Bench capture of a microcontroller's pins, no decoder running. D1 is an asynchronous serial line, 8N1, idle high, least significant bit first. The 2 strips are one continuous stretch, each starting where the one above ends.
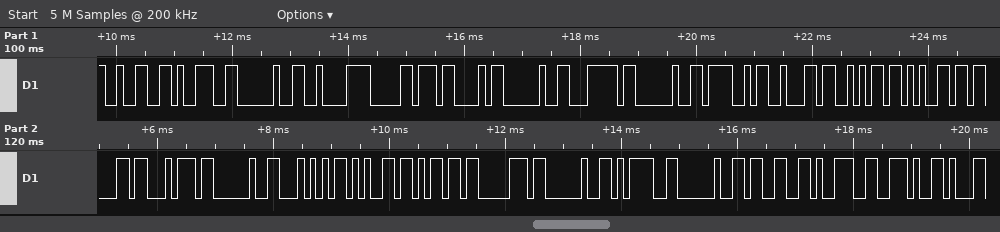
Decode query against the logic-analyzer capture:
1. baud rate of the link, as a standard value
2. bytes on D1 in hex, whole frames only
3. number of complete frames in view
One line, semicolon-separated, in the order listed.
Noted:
9600 baud; 0x32 0x39 0x20 0xC2 0xB0 0x43 0x20 0x7C 0x20 0x4F 0x62 0x6A 0x65 0x63 0x74 0x20 0x54 0x65 0x6D 0x70 0x20 0x3D 0x20 0x33 0x39 0x2E; 26
